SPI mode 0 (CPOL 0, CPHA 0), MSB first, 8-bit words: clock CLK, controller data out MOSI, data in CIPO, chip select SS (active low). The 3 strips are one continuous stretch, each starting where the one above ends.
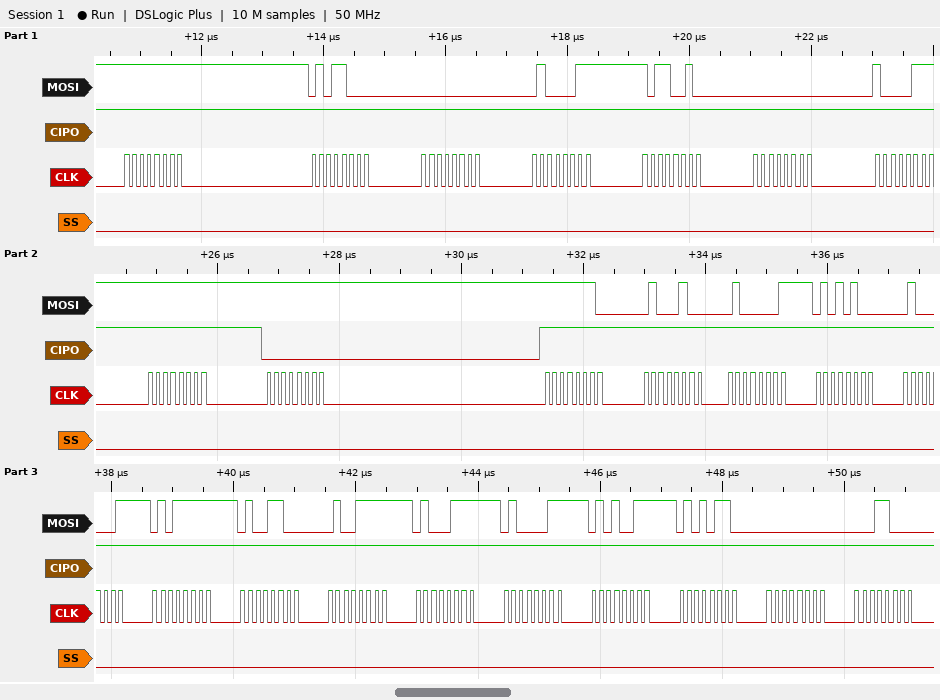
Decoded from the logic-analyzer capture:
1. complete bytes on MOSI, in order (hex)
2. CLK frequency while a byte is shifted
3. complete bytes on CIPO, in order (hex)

FF 58 00 43 B2 00 87 FF FF FE 44 41 54 41 5F 4C 4F 47 43 53 56 00 18
8 MHz
FF FF FF FF FF FF FF FF 00 FF FF FF FF FF FF FF FF FF FF FF FF FF FF
